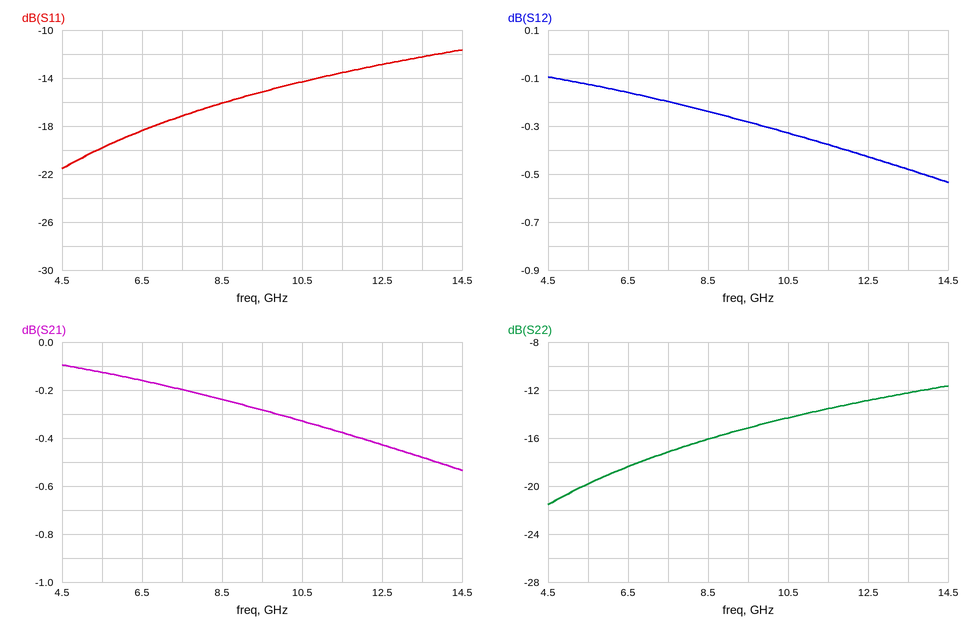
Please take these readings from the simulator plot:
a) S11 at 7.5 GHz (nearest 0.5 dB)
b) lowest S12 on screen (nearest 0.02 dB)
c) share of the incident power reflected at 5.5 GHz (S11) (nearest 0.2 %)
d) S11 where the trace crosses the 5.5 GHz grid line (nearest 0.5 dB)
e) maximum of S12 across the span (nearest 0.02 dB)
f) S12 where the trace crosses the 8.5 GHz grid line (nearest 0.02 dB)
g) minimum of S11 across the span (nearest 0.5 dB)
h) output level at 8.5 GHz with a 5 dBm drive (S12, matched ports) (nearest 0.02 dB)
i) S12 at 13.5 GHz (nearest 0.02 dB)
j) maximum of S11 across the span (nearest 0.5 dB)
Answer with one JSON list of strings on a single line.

["-17.0 dB", "-0.54 dB", "1.0 %", "-20.0 dB", "-0.10 dB", "-0.24 dB", "-21.5 dB", "4.76 dBm", "-0.48 dB", "-11.5 dB"]
